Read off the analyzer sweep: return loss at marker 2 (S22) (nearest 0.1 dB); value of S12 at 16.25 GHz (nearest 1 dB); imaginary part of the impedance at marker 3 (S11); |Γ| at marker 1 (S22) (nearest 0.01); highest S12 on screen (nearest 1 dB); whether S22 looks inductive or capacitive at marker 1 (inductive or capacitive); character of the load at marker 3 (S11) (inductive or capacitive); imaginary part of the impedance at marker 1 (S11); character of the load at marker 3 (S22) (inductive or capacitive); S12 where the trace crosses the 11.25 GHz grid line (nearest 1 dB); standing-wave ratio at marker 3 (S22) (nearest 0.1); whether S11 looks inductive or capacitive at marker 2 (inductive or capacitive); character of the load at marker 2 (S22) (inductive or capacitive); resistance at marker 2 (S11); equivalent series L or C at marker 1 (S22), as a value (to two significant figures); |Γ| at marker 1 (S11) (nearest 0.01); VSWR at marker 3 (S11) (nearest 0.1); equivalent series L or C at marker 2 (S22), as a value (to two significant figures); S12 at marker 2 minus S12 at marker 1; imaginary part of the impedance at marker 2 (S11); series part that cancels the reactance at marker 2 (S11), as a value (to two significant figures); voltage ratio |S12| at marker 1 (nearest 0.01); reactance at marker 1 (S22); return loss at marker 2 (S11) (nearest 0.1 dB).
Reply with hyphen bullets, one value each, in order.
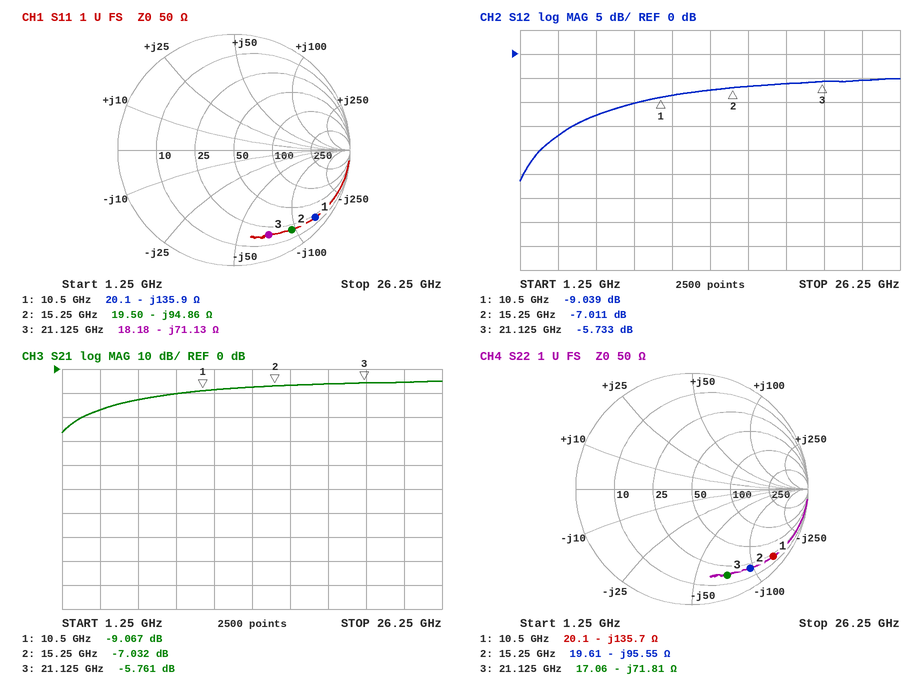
- 1.4 dB
- -7 dB
- -71.13 Ω
- 0.91
- -5 dB
- capacitive
- capacitive
- -135.9 Ω
- capacitive
- -9 dB
- 9.2
- capacitive
- capacitive
- 19.50 Ω
- 110 fF
- 0.91
- 8.6
- 110 fF
- 2.028 dB
- -94.86 Ω
- 990 pH
- 0.35
- -135.7 Ω
- 1.4 dB
